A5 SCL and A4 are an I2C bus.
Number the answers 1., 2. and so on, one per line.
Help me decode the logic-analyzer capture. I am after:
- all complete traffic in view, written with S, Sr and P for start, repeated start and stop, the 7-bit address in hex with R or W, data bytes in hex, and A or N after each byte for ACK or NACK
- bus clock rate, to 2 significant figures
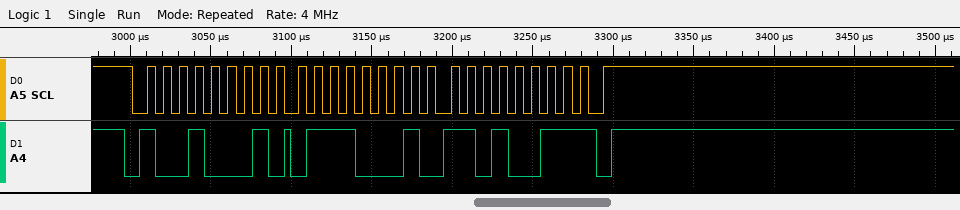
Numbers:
1. S 48R A 71 A D3 N P
2. 100 kHz
